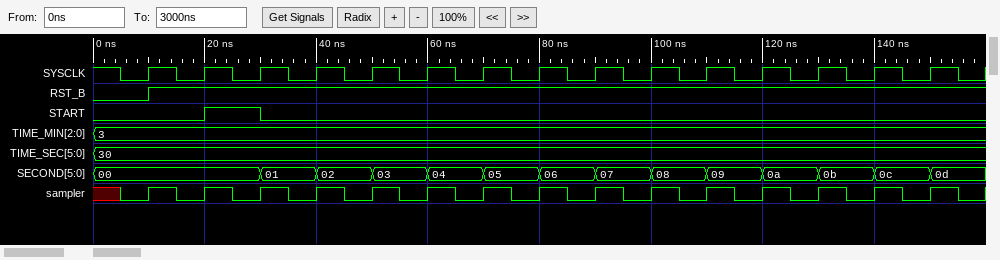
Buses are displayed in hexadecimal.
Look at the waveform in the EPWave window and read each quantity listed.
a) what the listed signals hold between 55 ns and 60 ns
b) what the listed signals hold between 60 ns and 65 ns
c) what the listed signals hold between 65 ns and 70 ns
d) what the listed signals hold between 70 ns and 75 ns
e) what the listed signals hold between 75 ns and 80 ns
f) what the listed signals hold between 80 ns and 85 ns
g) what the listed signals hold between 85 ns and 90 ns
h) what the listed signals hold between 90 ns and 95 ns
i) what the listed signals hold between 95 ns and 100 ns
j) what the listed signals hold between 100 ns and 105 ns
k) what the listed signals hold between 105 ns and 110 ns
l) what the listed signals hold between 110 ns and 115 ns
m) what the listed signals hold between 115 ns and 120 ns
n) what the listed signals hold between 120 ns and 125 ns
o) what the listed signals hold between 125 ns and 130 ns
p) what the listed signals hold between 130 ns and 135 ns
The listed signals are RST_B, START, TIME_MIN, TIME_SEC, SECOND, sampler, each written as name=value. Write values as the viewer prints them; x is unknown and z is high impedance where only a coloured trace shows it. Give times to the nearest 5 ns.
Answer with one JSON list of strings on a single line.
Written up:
["RST_B=1, START=0, TIME_MIN=3, TIME_SEC=30, SECOND=03, sampler=0", "RST_B=1, START=0, TIME_MIN=3, TIME_SEC=30, SECOND=04, sampler=1", "RST_B=1, START=0, TIME_MIN=3, TIME_SEC=30, SECOND=04, sampler=0", "RST_B=1, START=0, TIME_MIN=3, TIME_SEC=30, SECOND=05, sampler=1", "RST_B=1, START=0, TIME_MIN=3, TIME_SEC=30, SECOND=05, sampler=0", "RST_B=1, START=0, TIME_MIN=3, TIME_SEC=30, SECOND=06, sampler=1", "RST_B=1, START=0, TIME_MIN=3, TIME_SEC=30, SECOND=06, sampler=0", "RST_B=1, START=0, TIME_MIN=3, TIME_SEC=30, SECOND=07, sampler=1", "RST_B=1, START=0, TIME_MIN=3, TIME_SEC=30, SECOND=07, sampler=0", "RST_B=1, START=0, TIME_MIN=3, TIME_SEC=30, SECOND=08, sampler=1", "RST_B=1, START=0, TIME_MIN=3, TIME_SEC=30, SECOND=08, sampler=0", "RST_B=1, START=0, TIME_MIN=3, TIME_SEC=30, SECOND=09, sampler=1", "RST_B=1, START=0, TIME_MIN=3, TIME_SEC=30, SECOND=09, sampler=0", "RST_B=1, START=0, TIME_MIN=3, TIME_SEC=30, SECOND=0a, sampler=1", "RST_B=1, START=0, TIME_MIN=3, TIME_SEC=30, SECOND=0a, sampler=0", "RST_B=1, START=0, TIME_MIN=3, TIME_SEC=30, SECOND=0b, sampler=1"]
